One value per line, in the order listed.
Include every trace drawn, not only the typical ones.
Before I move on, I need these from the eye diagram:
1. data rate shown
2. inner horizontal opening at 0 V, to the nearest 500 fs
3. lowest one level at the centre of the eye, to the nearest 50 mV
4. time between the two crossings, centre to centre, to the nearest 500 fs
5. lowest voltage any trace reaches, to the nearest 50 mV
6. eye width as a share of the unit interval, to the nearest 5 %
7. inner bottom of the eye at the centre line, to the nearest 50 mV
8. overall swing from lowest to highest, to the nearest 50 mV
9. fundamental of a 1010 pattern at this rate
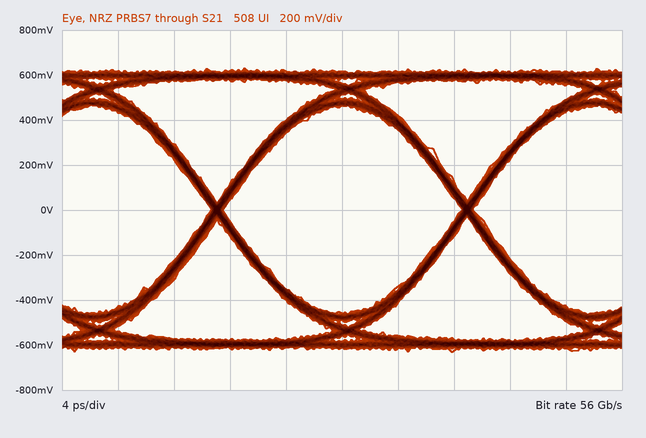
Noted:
56 Gb/s
17.0 ps
450 mV
18.0 ps
-650 mV
95 %
-450 mV
1.25 V
28 GHz
